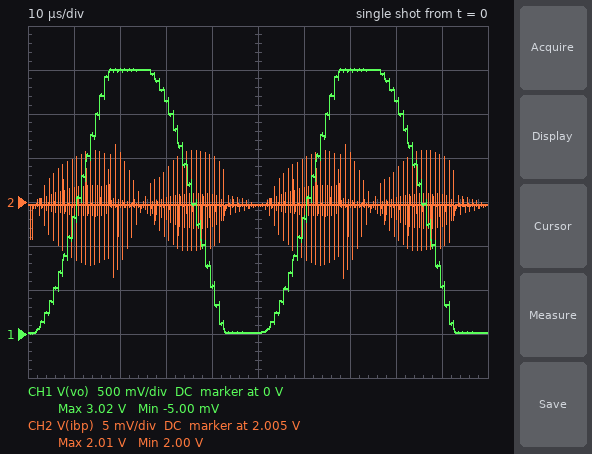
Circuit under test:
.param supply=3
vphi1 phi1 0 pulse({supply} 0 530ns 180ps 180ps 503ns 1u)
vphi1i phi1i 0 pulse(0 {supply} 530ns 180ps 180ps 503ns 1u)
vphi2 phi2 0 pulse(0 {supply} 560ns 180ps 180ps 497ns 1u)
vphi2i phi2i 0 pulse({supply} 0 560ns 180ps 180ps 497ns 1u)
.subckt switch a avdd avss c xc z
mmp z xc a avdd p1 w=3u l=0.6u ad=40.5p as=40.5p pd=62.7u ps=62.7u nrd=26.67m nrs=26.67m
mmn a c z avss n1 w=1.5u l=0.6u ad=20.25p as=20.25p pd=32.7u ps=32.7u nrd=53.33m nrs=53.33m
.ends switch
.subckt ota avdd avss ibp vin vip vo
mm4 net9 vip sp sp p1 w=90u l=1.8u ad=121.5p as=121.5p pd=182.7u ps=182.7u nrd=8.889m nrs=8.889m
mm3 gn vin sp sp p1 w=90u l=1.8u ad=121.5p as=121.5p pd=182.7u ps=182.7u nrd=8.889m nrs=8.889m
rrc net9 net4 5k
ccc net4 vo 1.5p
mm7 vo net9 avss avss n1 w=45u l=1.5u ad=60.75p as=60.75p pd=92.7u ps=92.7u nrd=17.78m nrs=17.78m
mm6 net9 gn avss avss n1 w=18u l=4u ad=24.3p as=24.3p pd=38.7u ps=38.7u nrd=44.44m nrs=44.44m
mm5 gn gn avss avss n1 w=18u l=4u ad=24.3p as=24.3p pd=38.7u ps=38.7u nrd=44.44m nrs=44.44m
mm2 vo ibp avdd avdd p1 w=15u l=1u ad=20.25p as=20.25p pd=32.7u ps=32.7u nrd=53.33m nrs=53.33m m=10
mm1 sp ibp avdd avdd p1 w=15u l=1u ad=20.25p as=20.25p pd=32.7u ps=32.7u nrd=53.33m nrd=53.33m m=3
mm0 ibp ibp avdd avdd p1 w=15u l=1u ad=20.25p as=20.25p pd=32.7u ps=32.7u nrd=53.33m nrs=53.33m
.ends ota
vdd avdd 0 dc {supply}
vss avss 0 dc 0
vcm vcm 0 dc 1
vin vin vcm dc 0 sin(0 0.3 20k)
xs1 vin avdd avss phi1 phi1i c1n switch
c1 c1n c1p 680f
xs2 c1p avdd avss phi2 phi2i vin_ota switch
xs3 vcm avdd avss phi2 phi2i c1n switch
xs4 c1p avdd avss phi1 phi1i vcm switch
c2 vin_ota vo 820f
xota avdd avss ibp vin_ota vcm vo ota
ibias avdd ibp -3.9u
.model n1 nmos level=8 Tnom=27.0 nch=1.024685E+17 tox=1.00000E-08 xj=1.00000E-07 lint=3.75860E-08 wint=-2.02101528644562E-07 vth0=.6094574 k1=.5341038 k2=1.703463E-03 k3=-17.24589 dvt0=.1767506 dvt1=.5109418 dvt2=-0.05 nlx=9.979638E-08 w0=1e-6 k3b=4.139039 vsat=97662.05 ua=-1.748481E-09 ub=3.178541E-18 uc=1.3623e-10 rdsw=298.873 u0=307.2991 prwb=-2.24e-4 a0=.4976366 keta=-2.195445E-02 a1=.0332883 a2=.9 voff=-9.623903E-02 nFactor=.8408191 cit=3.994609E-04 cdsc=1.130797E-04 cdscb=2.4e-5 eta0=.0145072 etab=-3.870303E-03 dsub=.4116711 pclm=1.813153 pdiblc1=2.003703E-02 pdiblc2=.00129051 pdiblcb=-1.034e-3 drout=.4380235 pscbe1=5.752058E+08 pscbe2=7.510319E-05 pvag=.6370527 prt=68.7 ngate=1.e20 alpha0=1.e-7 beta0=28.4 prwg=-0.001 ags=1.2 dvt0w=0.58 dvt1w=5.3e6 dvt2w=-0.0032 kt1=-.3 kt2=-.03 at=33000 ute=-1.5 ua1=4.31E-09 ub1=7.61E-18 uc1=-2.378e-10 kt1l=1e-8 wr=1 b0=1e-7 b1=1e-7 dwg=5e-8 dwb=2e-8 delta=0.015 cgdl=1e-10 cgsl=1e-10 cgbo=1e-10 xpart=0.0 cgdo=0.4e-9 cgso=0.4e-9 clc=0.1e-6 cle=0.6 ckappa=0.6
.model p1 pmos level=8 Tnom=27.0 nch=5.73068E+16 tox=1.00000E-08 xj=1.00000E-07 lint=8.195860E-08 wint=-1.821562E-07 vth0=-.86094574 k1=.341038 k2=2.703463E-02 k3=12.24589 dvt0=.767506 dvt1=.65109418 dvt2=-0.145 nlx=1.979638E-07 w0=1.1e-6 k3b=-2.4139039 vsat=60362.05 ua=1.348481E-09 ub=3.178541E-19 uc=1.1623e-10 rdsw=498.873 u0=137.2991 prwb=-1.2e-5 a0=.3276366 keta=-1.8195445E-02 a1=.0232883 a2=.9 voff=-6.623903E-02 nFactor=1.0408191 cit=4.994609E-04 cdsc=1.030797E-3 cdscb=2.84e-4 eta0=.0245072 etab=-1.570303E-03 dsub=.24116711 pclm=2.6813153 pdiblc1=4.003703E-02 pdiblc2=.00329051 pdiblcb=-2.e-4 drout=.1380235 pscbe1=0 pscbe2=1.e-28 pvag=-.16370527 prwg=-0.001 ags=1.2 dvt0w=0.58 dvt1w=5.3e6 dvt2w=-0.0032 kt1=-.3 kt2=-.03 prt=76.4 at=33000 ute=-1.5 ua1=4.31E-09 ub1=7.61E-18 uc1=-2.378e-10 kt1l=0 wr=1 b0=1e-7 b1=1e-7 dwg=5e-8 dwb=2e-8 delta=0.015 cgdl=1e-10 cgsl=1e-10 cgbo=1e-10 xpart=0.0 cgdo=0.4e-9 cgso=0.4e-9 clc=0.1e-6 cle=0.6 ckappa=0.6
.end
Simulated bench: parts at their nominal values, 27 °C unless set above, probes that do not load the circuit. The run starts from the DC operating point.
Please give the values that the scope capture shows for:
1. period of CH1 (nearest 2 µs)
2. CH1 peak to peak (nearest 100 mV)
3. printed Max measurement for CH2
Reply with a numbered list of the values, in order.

1. 50 µs
2. 3.0 V
3. 2.01 V
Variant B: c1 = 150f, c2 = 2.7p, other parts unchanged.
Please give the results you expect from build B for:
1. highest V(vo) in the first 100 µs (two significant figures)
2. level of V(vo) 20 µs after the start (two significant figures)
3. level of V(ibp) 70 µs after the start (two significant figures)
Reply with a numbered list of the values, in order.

1. 290 mV
2. 230 mV
3. 2.0 V
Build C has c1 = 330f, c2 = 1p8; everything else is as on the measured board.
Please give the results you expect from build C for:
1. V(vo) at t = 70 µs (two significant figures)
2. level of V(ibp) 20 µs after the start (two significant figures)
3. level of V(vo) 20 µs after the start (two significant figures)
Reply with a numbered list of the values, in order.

1. 770 mV
2. 2.0 V
3. 730 mV
